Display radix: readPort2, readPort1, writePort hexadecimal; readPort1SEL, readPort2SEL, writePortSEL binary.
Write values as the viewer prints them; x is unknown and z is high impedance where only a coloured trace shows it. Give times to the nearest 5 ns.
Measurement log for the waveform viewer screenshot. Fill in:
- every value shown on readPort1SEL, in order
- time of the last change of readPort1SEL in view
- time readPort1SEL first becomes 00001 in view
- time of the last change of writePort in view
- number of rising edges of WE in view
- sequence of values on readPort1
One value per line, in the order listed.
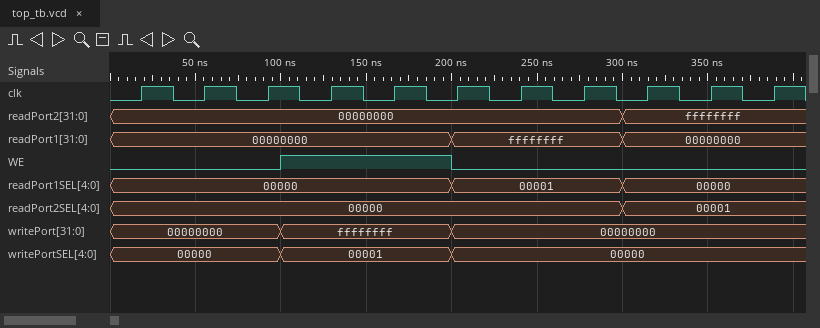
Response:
00000, 00001, 00000
300 ns
200 ns
200 ns
1
00000000, ffffffff, 00000000
